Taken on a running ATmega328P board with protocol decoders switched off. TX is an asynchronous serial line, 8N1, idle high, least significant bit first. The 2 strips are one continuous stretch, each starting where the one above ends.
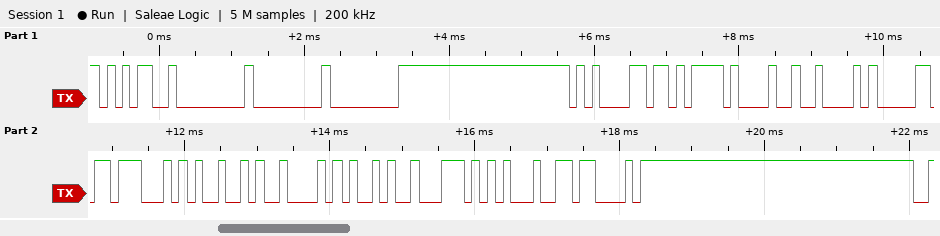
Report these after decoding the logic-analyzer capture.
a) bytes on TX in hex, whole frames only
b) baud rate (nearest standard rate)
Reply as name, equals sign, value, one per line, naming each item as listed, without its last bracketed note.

bytes on TX in hex, whole frames only = 0x35 0x00 0x00 0x00 0x85 0xEB 0x21 0x42 0xB0 0x47 0x49 0x42 0x29 0x5C 0x91 0x43
baud rate = 9600 baud
